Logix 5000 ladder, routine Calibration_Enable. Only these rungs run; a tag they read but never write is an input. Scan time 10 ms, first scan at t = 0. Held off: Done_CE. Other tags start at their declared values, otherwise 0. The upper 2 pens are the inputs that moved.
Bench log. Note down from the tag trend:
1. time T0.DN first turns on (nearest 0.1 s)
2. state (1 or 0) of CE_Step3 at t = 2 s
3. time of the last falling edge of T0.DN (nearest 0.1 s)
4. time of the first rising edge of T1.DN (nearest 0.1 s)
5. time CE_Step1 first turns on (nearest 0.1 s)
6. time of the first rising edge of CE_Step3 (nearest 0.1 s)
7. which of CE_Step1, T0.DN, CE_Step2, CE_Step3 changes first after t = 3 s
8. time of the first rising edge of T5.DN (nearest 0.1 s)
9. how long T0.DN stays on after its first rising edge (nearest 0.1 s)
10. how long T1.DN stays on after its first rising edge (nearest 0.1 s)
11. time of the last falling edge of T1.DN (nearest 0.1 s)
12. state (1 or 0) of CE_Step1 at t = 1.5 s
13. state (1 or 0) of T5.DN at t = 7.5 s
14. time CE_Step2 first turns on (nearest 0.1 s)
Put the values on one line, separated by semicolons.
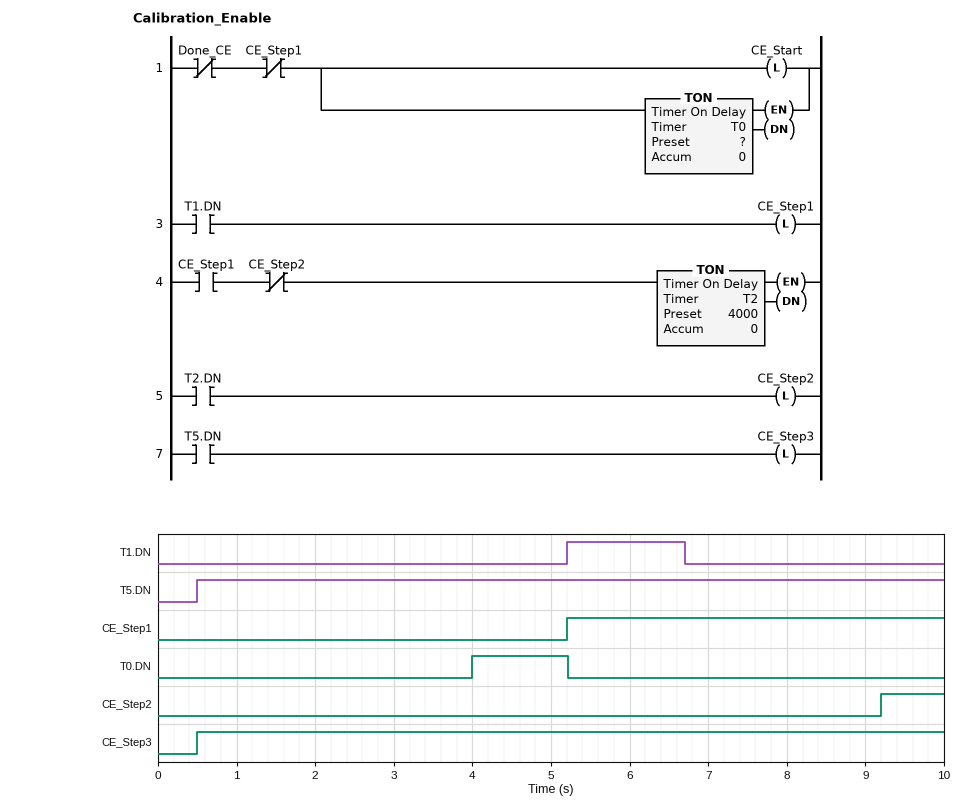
4.0 s; 1; 5.2 s; 5.2 s; 5.2 s; 0.5 s; T0.DN; 0.5 s; 1.2 s; 1.5 s; 6.7 s; 0; 1; 9.2 s
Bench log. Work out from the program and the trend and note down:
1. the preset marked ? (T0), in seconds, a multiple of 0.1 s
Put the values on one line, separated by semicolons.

4.0 s
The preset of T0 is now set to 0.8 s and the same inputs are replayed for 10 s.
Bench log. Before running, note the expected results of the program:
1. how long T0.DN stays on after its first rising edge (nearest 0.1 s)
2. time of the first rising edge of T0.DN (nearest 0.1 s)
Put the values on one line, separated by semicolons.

4.4 s; 0.8 s
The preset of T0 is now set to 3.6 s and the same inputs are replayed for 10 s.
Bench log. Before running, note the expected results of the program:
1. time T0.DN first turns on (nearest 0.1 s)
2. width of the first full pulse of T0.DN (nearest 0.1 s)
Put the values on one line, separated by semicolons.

3.6 s; 1.6 s
